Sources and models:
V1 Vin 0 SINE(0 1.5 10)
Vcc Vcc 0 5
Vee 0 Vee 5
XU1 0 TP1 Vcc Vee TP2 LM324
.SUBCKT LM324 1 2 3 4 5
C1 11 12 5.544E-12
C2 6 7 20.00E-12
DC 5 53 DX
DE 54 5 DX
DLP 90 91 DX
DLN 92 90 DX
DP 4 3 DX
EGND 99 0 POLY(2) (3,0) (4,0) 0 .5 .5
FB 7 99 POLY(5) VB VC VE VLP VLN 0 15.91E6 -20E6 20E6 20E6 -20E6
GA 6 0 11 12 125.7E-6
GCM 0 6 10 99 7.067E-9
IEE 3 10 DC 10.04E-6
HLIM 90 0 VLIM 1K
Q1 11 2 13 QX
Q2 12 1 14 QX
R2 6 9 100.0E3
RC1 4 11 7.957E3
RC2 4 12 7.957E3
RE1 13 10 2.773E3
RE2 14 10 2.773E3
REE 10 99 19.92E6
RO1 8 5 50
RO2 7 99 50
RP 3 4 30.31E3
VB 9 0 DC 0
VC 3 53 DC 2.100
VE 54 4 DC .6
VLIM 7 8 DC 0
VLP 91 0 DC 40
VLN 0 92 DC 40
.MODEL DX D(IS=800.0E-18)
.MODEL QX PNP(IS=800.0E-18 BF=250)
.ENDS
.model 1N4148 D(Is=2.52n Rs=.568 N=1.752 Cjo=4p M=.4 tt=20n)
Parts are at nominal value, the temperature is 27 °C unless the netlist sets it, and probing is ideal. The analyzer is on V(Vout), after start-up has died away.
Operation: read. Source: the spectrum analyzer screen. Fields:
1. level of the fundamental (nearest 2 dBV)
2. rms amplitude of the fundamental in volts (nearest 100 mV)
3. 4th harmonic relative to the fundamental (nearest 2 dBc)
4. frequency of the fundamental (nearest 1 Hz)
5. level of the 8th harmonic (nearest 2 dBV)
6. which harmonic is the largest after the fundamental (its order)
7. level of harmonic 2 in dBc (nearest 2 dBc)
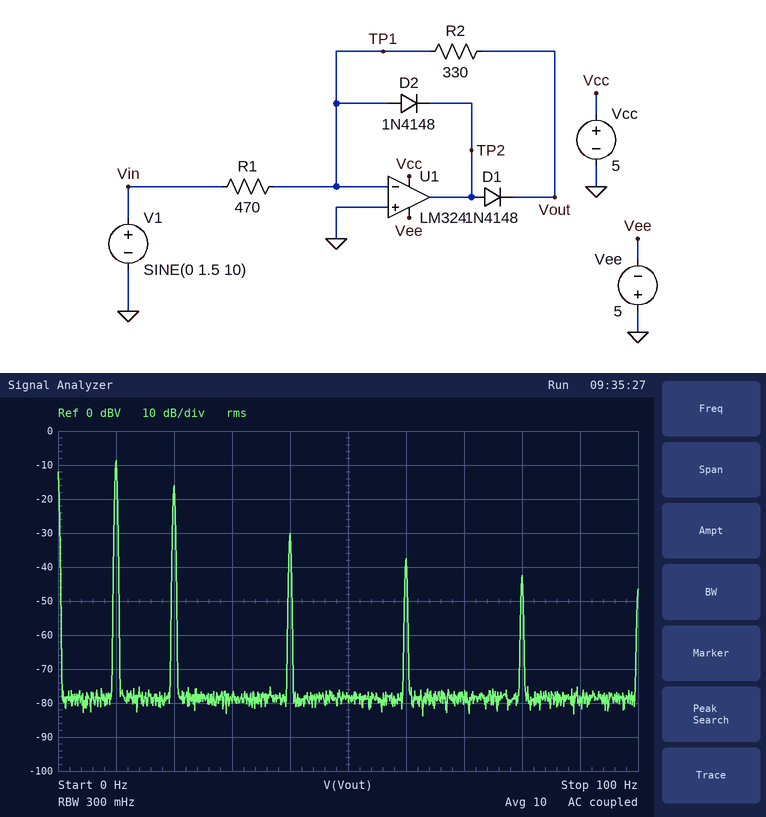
-8 dBV
400 mV
-22 dBc
10 Hz
-42 dBV
2
-8 dBc
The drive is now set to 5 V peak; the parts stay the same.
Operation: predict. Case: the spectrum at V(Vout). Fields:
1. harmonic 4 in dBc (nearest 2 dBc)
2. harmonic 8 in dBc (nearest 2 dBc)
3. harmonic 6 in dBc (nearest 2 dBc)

-16 dBc
-36 dBc
-32 dBc
